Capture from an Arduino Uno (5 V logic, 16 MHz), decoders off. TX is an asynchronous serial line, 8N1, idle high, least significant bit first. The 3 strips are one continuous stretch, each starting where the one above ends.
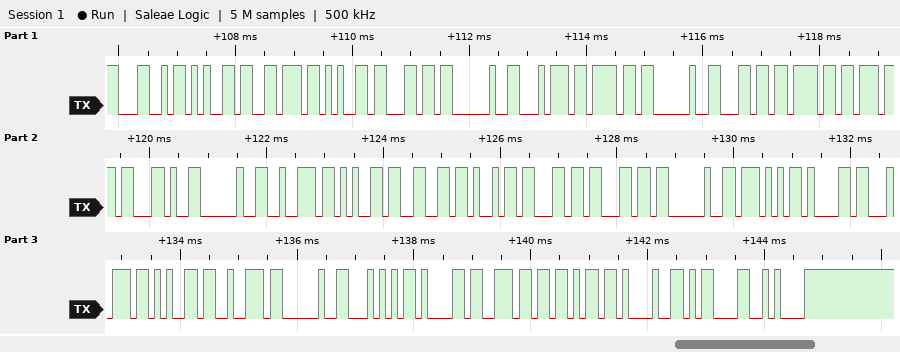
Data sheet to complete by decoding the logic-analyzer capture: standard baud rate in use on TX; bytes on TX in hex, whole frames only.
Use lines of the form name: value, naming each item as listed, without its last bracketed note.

standard baud rate in use on TX: 9600 baud
bytes on TX in hex, whole frames only: 0x4C 0x65 0x76 0x65 0x6C 0x20 0x74 0x6F 0x20 0x6C 0x6F 0x77 0x2C 0x20 0x72 0x65 0x66 0x69 0x6C 0x6C 0x20 0x57 0x61 0x74 0x65 0x72 0x20 0x54 0x61 0x6E 0x6B 0x21 0x0D 0x0A
